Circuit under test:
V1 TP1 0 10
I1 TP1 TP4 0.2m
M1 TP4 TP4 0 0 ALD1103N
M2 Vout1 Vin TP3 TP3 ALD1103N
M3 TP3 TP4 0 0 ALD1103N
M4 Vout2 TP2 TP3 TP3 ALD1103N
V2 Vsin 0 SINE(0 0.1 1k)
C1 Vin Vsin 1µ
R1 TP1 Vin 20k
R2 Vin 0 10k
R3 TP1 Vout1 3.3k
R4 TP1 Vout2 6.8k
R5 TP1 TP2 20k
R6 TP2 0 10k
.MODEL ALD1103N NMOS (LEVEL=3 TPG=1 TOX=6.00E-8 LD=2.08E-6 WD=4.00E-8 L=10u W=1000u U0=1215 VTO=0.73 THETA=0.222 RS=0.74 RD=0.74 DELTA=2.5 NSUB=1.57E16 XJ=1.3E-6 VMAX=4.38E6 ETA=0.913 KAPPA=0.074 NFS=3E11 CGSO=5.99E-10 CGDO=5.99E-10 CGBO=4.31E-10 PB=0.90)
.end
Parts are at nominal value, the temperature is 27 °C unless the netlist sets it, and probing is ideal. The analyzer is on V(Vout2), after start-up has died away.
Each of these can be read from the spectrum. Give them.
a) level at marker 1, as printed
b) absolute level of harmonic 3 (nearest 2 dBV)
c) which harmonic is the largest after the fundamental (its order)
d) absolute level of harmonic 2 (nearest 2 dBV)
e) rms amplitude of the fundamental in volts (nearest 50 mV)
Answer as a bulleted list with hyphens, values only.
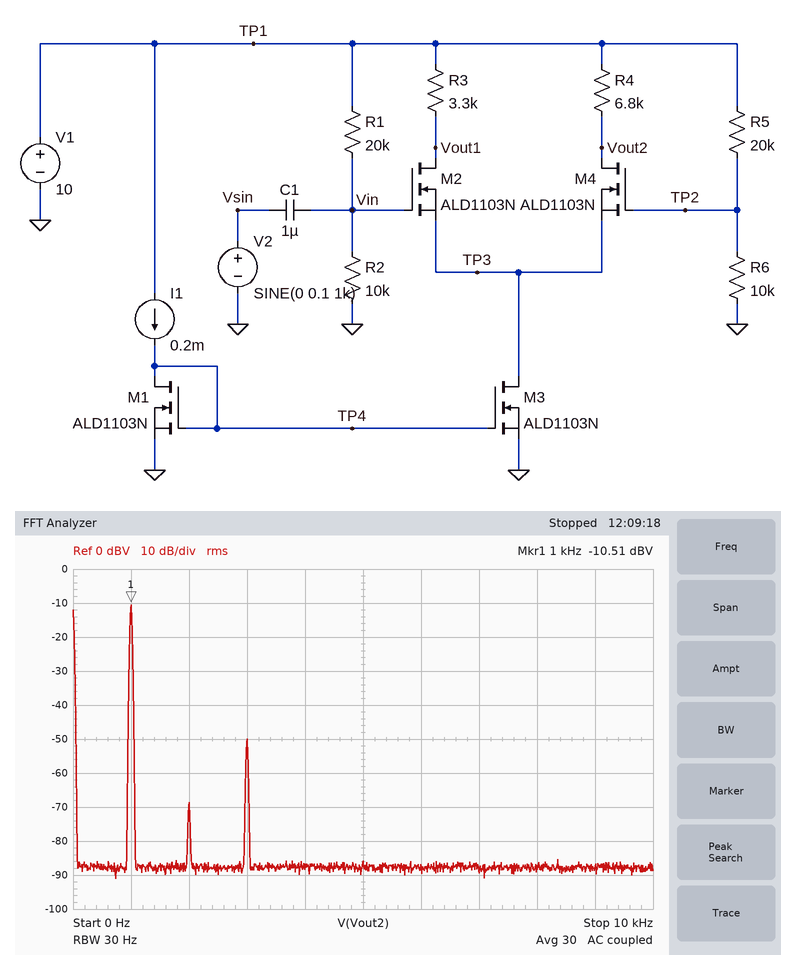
- -10.51 dBV
- -50 dBV
- 3
- -68 dBV
- 300 mV
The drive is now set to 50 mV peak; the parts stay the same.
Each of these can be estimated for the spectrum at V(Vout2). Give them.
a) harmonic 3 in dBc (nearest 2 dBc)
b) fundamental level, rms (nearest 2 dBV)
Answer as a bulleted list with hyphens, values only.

- -52 dBc
- -16 dBV
